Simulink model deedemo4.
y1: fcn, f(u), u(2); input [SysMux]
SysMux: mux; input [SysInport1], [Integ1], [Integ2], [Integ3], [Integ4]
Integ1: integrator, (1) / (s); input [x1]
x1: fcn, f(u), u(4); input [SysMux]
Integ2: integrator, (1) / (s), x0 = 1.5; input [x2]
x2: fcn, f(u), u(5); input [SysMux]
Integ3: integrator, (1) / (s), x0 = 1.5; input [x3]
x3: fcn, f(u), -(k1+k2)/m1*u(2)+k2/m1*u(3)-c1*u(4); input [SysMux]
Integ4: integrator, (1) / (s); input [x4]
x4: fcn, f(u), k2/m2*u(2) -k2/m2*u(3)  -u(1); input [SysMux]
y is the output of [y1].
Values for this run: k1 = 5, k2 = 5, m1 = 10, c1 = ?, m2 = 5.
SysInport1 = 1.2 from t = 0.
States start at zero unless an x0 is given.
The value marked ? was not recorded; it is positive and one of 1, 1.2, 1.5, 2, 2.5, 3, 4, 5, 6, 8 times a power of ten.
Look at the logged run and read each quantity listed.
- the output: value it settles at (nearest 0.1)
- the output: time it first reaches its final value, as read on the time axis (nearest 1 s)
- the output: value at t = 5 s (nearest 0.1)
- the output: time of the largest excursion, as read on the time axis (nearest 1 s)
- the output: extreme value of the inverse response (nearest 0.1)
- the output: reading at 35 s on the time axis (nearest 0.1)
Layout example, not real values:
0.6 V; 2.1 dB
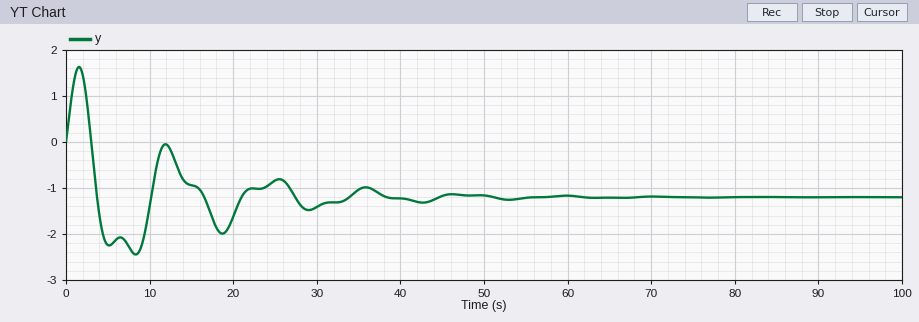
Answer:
-1.2; 4 s; -2.2; 8 s; 1.6; -1.0
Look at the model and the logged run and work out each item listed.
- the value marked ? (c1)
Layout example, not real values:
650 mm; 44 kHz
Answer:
0.3
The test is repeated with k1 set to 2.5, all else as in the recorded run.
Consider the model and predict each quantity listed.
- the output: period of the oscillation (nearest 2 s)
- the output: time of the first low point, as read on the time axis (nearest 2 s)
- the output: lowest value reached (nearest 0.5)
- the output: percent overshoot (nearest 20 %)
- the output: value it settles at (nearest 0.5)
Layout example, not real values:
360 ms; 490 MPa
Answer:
16 s; 10 s; -4.5; 100 %; -2.5
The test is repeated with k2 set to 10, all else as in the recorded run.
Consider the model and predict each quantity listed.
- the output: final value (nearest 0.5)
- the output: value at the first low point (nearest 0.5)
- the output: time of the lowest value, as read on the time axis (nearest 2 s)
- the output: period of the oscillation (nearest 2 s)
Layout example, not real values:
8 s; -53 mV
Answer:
-1.0; -3.0; 6 s; 10 s
